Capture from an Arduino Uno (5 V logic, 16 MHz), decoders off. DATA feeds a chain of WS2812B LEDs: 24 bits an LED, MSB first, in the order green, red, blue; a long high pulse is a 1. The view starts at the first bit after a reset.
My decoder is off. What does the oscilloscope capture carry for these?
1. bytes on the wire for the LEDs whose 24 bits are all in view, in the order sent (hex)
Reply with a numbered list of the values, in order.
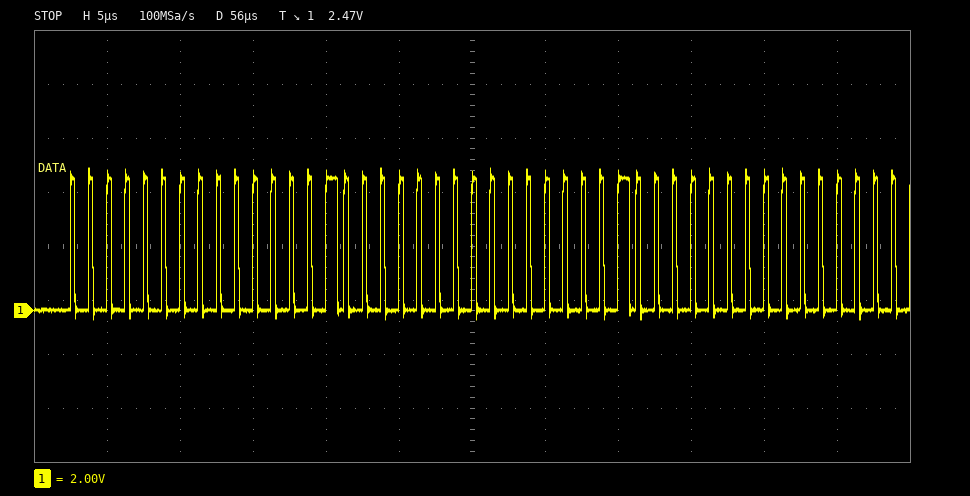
1. 00 02 00
